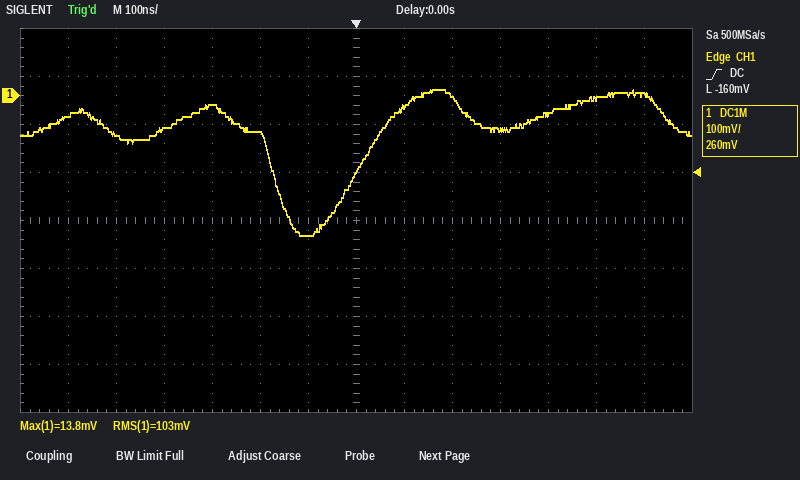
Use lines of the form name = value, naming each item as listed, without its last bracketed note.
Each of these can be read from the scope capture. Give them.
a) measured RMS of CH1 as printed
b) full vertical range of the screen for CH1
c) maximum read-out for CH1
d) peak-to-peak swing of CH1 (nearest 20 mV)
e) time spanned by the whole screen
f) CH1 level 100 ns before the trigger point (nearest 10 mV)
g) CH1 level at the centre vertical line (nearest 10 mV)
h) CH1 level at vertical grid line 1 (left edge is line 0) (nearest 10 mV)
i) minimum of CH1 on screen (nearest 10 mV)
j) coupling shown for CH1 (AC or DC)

measured RMS of CH1 as printed = 103 mV
full vertical range of the screen for CH1 = 800 mV
maximum read-out for CH1 = 13.8 mV
peak-to-peak swing of CH1 = 300 mV
time spanned by the whole screen = 1.4 µs
CH1 level 100 ns before the trigger point = -290 mV
CH1 level at the centre vertical line = -160 mV
CH1 level at vertical grid line 1 (left edge is line 0) = -40 mV
minimum of CH1 on screen = -290 mV
coupling shown for CH1 = DC
